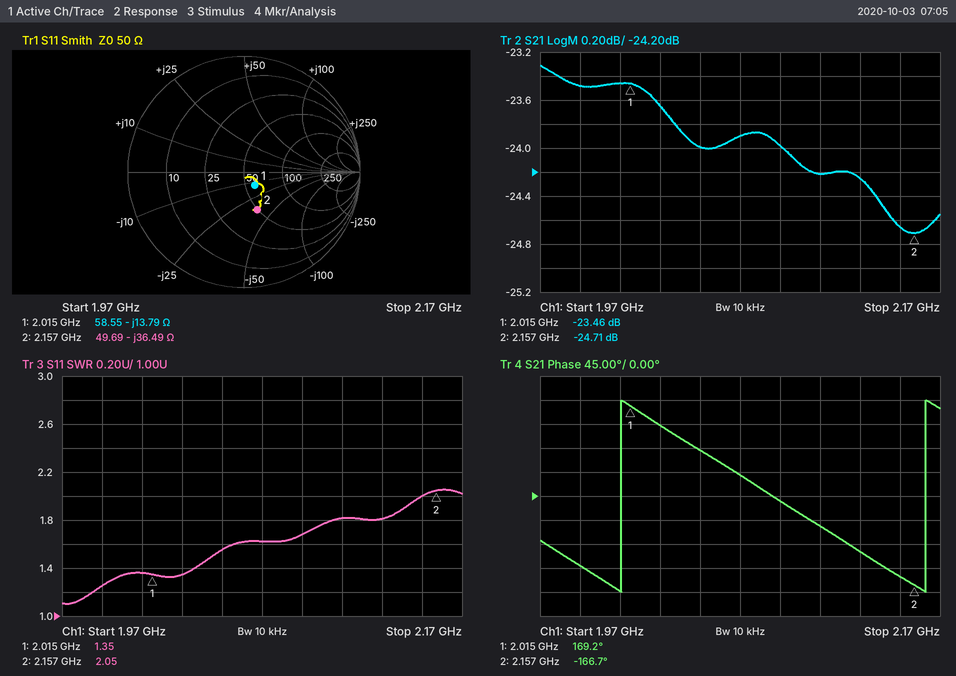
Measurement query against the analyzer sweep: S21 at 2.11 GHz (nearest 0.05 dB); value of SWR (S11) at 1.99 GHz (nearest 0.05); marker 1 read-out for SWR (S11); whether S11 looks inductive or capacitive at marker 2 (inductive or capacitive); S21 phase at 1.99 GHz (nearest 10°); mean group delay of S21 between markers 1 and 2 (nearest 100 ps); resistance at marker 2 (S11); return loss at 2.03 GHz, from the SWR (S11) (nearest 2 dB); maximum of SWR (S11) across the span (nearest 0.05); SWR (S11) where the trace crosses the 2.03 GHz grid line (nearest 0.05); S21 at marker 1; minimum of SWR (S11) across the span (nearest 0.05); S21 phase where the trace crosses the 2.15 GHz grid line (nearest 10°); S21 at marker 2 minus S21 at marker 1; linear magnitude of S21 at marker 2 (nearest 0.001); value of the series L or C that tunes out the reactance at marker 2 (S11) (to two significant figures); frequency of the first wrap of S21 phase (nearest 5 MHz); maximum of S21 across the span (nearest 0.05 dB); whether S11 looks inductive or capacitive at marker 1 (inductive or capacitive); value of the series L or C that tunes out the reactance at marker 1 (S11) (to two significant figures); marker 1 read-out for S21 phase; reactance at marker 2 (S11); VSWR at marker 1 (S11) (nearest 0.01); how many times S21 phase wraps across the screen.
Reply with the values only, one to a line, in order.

-24.20 dB
1.25
1.35
capacitive
-130°
6.6 ns
49.69 Ω
16 dB
2.05
1.35
-23.46 dB
1.10
-150°
-1.25 dB
0.058
2.7 nH
2.010 GHz
-23.30 dB
capacitive
1.1 nH
169.2°
-36.49 Ω
1.35
2
